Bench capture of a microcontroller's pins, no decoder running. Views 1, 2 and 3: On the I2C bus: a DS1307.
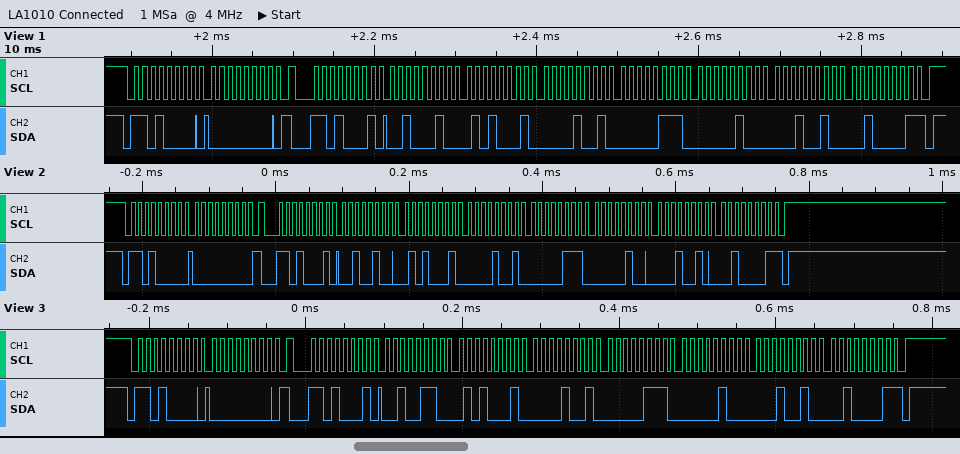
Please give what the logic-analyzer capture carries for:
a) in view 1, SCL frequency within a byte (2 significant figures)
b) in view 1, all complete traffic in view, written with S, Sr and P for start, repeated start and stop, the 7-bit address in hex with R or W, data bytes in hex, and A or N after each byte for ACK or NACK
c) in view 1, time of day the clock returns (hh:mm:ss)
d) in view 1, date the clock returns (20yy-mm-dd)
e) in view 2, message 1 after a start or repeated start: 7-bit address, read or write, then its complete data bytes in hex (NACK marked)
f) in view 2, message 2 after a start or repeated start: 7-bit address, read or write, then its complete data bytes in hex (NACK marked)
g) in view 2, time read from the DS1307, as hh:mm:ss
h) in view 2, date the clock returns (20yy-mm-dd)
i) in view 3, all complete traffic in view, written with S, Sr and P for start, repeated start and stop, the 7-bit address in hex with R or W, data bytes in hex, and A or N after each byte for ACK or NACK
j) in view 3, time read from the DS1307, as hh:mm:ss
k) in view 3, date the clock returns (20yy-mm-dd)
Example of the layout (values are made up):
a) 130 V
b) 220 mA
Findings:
a) 100 kHz
b) S 68W A 00 A Sr 68R A 22 A 51 A 09 A 07 A 04 A 12 A 21 N P
c) 09:51:22
d) 2021-12-04
e) 0x68 write: 00
f) 0x68 read: 24 51 09 07 04 12 21 NACK
g) 09:51:24
h) 2021-12-04
i) S 68W A 00 A Sr 68R A 26 A 51 A 09 A 07 A 04 A 12 A 21 N P
j) 09:51:26
k) 2021-12-04
